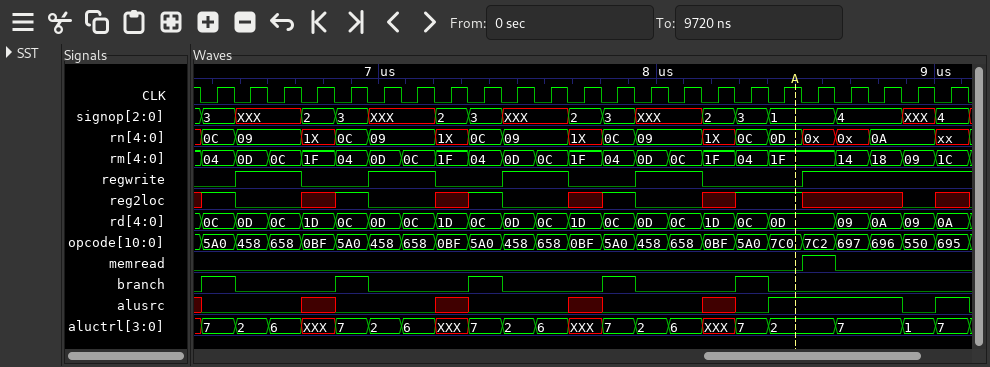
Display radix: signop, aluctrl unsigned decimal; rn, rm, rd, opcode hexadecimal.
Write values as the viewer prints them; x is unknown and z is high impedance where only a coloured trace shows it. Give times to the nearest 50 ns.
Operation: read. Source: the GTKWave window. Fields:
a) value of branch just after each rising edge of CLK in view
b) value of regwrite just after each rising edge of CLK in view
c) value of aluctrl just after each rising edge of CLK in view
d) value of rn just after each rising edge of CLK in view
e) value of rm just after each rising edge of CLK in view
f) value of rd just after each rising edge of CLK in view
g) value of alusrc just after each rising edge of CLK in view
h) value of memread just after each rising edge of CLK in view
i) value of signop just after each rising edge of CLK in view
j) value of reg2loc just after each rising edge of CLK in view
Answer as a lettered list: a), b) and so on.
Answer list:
a) 1 0 0 0 1 0 0 0 1 0 0 0 1 0 0 0 1 0 0 0 0 0 0
b) 0 1 1 0 0 1 1 0 0 1 1 0 0 1 1 0 0 0 1 1 1 1 1
c) 7, 2, 6, XXX, 7, 2, 6, XXX, 7, 2, 6, XXX, 7, 2, 6, XXX, 7, 2, 2, 7, 7, 1, 7
d) 0C, 09, 09, 1X, 0C, 09, 09, 1X, 0C, 09, 09, 1X, 0C, 09, 09, 1X, 0C, 0D, 0x, 0x, 0A, 0A, xx
e) 04, 0D, 0C, 1F, 04, 0D, 0C, 1F, 04, 0D, 0C, 1F, 04, 0D, 0C, 1F, 04, 1F, 1F, 14, 18, 09, 1C
f) 0C, 0D, 0C, 1D, 0C, 0D, 0C, 1D, 0C, 0D, 0C, 1D, 0C, 0D, 0C, 1D, 0C, 0D, 0D, 09, 0A, 09, 0A
g) 0 0 0 x 0 0 0 x 0 0 0 x 0 0 0 x 0 1 1 1 1 0 1
h) 0 0 0 0 0 0 0 0 0 0 0 0 0 0 0 0 0 0 1 0 0 0 0
i) 3, XXX, XXX, 2, 3, XXX, XXX, 2, 3, XXX, XXX, 2, 3, XXX, XXX, 2, 3, 1, 1, 4, 4, XXX, 4
j) 1 0 0 x 1 0 0 x 1 0 0 x 1 0 0 x 1 1 x x x 0 x
